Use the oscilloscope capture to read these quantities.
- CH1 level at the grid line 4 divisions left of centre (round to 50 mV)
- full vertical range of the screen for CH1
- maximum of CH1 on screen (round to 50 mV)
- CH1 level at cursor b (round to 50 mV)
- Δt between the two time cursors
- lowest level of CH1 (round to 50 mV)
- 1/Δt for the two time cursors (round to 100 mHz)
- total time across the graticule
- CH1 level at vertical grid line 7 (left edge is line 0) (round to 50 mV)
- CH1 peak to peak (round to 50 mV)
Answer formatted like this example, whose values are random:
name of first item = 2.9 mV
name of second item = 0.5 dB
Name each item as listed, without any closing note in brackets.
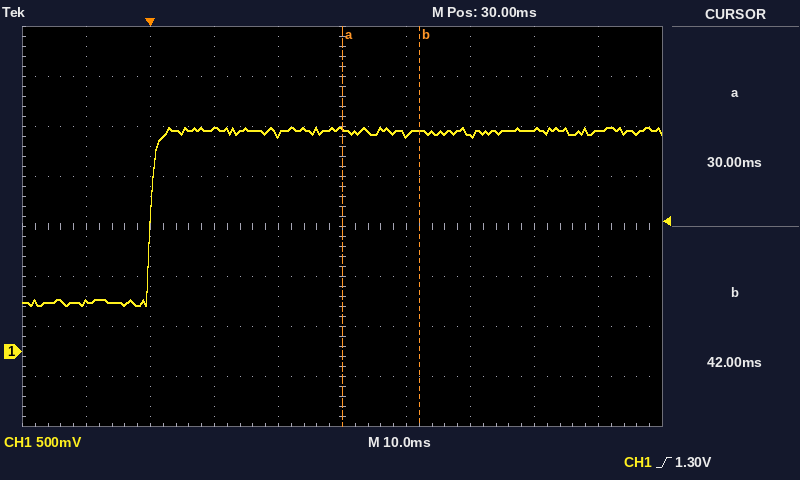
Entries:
CH1 level at the grid line 4 divisions left of centre = 500 mV
full vertical range of the screen for CH1 = 4 V
maximum of CH1 on screen = 2.25 V
CH1 level at cursor b = 2.20 V
Δt between the two time cursors = 12 ms
lowest level of CH1 = 450 mV
1/Δt for the two time cursors = 83.3 Hz
total time across the graticule = 100 ms
CH1 level at vertical grid line 7 (left edge is line 0) = 2.15 V
CH1 peak to peak = 1.80 V
